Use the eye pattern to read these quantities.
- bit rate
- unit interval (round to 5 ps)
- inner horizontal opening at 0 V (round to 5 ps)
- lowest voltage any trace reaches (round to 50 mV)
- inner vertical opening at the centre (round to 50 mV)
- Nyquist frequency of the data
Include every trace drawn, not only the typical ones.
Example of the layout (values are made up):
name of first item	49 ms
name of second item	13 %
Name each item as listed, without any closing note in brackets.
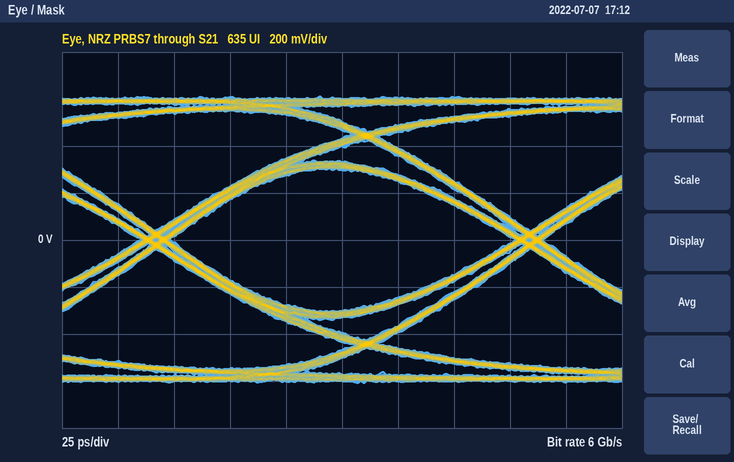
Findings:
bit rate	6 Gb/s
unit interval	165 ps
inner horizontal opening at 0 V	155 ps
lowest voltage any trace reaches	-600 mV
inner vertical opening at the centre	600 mV
Nyquist frequency of the data	3 GHz
